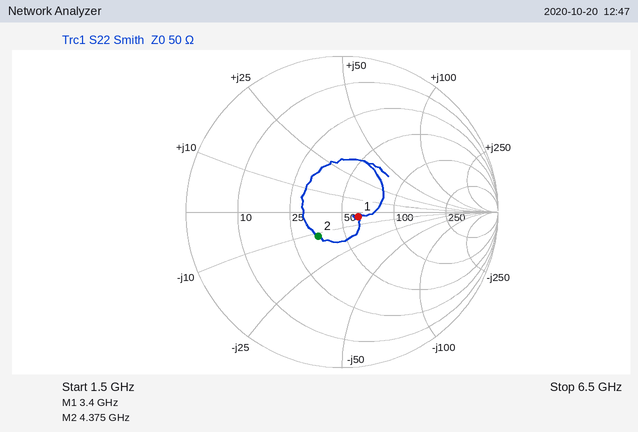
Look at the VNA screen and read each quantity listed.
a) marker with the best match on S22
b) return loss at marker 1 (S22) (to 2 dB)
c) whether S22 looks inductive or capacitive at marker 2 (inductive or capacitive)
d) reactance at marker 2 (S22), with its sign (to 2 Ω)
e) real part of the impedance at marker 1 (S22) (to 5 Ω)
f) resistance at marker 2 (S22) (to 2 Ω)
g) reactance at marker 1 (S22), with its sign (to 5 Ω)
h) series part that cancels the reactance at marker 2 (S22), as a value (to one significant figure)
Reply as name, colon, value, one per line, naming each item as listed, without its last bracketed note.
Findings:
marker with the best match on S22: marker 1
return loss at marker 1 (S22): 20 dB
whether S22 looks inductive or capacitive at marker 2: capacitive
reactance at marker 2 (S22), with its sign: -12 Ω
real part of the impedance at marker 1 (S22): 60 Ω
resistance at marker 2 (S22): 36 Ω
reactance at marker 1 (S22), with its sign: -5 Ω
series part that cancels the reactance at marker 2 (S22), as a value: 400 pH
